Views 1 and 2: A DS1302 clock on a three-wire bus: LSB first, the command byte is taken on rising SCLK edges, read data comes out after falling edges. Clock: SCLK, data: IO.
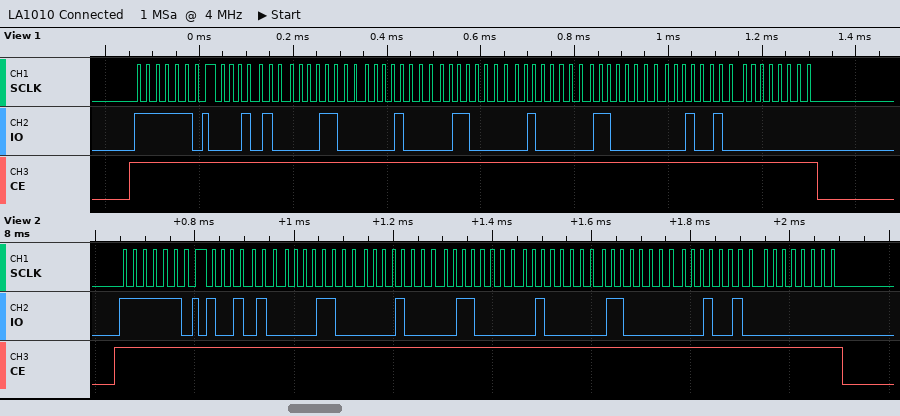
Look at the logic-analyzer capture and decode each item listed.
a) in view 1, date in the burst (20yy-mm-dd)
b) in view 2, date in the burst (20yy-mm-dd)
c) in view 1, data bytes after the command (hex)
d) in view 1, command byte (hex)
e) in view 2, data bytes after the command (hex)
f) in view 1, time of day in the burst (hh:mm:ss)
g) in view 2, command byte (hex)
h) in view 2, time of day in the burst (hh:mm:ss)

2024-02-06
2024-02-06
28 18 08 06 02 03 24 00
0xBF
29 18 08 06 02 03 24 00
08:18:28
0xBF
08:18:29
